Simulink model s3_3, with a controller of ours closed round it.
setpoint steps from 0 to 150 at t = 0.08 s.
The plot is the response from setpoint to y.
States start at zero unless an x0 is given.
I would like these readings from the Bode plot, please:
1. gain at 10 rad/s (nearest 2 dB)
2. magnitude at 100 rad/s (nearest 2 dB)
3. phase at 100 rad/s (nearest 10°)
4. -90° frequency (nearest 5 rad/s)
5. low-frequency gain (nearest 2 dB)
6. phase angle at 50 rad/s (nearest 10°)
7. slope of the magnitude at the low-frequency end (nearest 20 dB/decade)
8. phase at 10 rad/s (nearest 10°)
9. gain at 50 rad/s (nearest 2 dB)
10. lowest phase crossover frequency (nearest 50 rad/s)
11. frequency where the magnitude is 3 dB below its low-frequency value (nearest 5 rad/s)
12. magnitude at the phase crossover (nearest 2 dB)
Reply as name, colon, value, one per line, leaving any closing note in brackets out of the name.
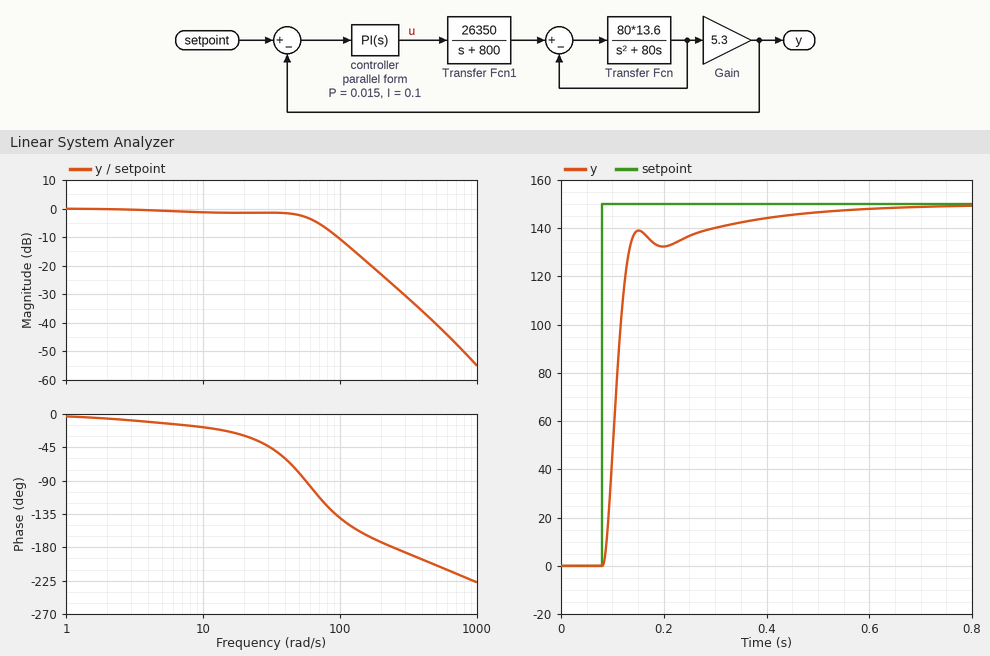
gain at 10 rad/s: -2 dB
magnitude at 100 rad/s: -10 dB
phase at 100 rad/s: -140°
-90° frequency: 55 rad/s
low-frequency gain: 0 dB
phase angle at 50 rad/s: -80°
slope of the magnitude at the low-frequency end: 0 dB/decade
phase at 10 rad/s: -20°
gain at 50 rad/s: -2 dB
lowest phase crossover frequency: 250 rad/s
frequency where the magnitude is 3 dB below its low-frequency value: 55 rad/s
magnitude at the phase crossover: -26 dB
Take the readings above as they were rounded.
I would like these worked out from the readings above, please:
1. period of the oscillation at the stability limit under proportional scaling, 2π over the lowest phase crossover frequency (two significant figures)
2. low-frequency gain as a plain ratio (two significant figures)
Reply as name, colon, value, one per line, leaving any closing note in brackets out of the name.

period of the oscillation at the stability limit under proportional scaling, 2π over the lowest phase crossover frequency: 0.025 s
low-frequency gain as a plain ratio: 1.0
